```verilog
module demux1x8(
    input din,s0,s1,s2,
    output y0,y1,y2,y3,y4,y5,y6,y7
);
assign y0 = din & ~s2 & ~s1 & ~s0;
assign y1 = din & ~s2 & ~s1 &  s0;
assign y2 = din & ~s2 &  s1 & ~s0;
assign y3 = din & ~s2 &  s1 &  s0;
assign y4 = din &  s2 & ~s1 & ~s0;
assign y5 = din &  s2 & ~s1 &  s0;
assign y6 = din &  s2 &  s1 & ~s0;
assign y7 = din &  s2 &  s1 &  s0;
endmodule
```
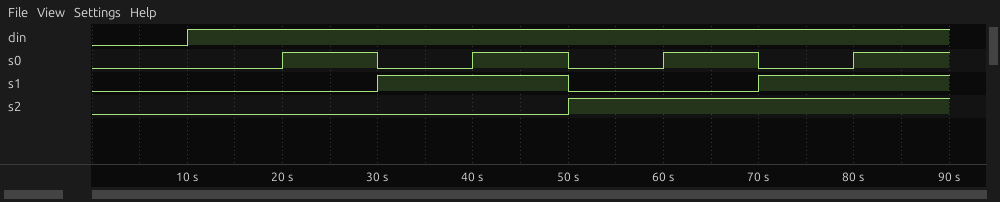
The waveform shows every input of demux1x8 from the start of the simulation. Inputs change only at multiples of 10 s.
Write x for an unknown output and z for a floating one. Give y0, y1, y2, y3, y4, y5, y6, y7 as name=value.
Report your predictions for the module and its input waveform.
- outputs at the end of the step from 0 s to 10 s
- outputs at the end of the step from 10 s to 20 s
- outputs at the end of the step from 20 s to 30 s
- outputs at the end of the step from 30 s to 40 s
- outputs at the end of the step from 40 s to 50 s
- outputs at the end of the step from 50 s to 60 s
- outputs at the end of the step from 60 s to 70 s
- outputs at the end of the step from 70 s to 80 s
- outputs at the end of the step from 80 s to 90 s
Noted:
y0=0, y1=0, y2=0, y3=0, y4=0, y5=0, y6=0, y7=0
y0=1, y1=0, y2=0, y3=0, y4=0, y5=0, y6=0, y7=0
y0=0, y1=1, y2=0, y3=0, y4=0, y5=0, y6=0, y7=0
y0=0, y1=0, y2=1, y3=0, y4=0, y5=0, y6=0, y7=0
y0=0, y1=0, y2=0, y3=1, y4=0, y5=0, y6=0, y7=0
y0=0, y1=0, y2=0, y3=0, y4=1, y5=0, y6=0, y7=0
y0=0, y1=0, y2=0, y3=0, y4=0, y5=1, y6=0, y7=0
y0=0, y1=0, y2=0, y3=0, y4=0, y5=0, y6=1, y7=0
y0=0, y1=0, y2=0, y3=0, y4=0, y5=0, y6=0, y7=1
